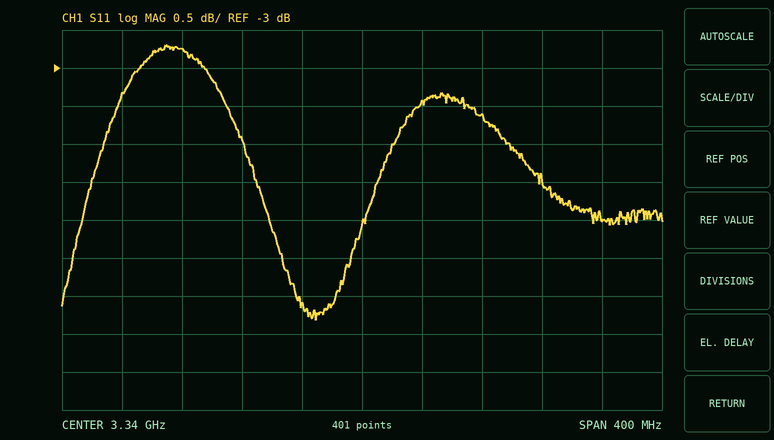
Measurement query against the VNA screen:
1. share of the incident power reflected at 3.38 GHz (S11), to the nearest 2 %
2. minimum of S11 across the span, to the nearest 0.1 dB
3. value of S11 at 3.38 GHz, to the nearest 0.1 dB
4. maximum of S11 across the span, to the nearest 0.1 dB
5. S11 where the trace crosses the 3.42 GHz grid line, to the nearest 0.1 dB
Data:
46 %
-6.3 dB
-3.4 dB
-2.7 dB
-3.6 dB
